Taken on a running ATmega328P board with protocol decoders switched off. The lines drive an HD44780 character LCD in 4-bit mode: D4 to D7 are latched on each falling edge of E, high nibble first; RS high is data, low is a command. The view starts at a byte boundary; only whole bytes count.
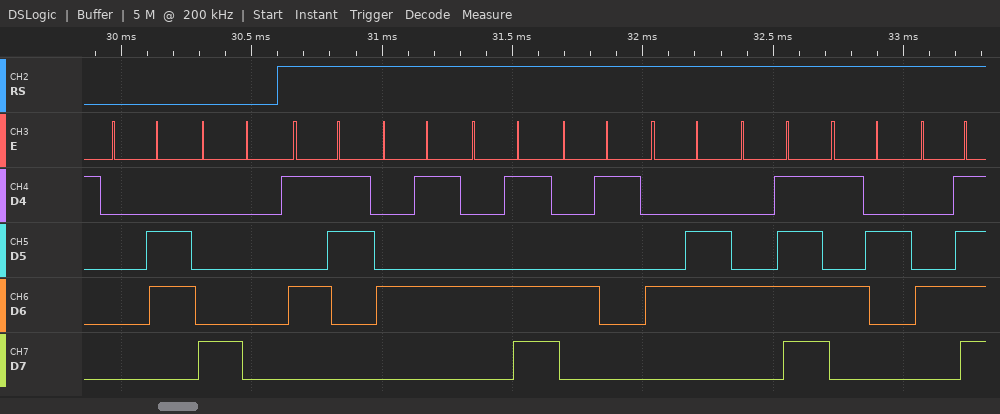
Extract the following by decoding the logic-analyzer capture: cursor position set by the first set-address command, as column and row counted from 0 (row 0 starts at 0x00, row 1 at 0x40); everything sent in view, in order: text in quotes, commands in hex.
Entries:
column 0, row 0
0x06 0x80 "SEMAFORO"
